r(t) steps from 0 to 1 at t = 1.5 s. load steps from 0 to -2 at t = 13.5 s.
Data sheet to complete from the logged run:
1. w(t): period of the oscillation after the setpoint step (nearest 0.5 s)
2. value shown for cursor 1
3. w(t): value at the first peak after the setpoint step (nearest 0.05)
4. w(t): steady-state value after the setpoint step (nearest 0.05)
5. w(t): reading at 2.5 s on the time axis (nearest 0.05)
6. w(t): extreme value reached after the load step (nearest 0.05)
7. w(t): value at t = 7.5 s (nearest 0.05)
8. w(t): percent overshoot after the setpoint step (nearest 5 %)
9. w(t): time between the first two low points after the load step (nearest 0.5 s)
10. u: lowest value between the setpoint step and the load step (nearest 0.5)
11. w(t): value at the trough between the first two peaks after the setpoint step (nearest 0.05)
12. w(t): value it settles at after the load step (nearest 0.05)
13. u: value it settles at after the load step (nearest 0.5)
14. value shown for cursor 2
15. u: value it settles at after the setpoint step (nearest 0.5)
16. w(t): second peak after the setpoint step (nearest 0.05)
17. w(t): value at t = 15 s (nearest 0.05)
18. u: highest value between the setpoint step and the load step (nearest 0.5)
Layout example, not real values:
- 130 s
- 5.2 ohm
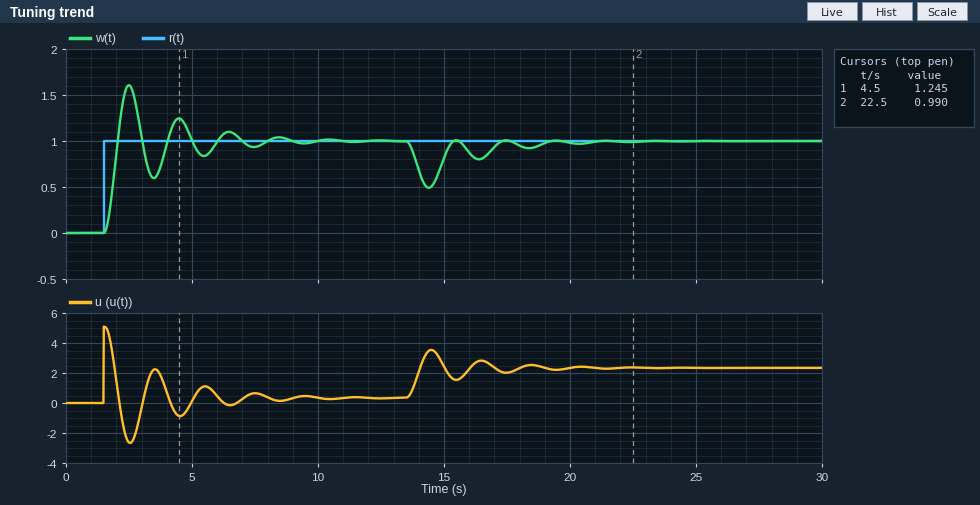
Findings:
- 2.0 s
- 1.245
- 1.60
- 1.00
- 1.60
- 0.50
- 0.95
- 60 %
- 2.0 s
- -2.5
- 0.60
- 1.00
- 2.5
- 0.990
- 0.5
- 1.25
- 0.80
- 5.0
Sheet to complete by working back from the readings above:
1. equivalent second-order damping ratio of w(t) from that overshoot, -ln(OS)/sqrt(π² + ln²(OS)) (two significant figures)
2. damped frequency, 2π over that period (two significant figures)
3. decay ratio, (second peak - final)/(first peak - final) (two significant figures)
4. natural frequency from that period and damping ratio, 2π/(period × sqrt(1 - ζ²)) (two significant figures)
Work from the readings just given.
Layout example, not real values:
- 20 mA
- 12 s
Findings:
- 0.16
- 3.1 rad/s
- 0.42
- 3.2 rad/s
